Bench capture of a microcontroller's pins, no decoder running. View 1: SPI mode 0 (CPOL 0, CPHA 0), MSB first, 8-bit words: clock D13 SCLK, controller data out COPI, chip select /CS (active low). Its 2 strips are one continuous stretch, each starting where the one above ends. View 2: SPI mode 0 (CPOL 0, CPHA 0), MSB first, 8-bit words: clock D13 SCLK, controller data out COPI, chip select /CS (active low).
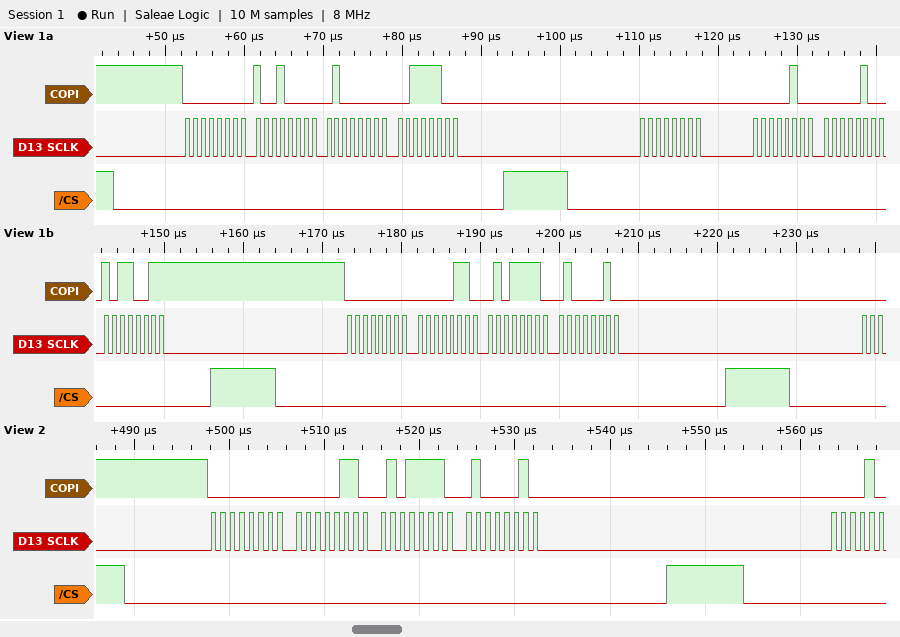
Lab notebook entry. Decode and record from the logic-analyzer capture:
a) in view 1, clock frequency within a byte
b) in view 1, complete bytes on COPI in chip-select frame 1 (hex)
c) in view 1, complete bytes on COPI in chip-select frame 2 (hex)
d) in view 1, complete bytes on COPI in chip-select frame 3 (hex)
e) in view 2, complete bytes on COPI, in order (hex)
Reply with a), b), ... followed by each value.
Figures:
a) 1 MHz
b) 00 90 40 3C
c) 00 04 04 B3
d) 00 06 5E 42
e) 0x00 0x06 0x5E 0x42
